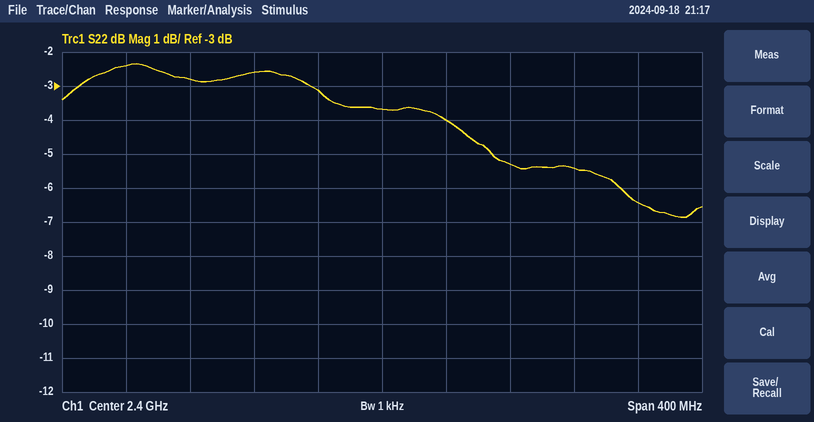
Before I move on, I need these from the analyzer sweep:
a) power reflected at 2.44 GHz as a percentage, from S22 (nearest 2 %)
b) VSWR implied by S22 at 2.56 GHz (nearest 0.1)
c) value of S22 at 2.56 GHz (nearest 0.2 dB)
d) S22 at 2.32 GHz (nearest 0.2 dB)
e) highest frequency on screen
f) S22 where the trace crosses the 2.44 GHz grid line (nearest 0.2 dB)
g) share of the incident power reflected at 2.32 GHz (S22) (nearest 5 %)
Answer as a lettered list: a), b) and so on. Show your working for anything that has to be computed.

a) 10^(-4/10) ≈ 40 %
b) |Γ| = 10^(-6.4/20) = 0.4786; VSWR = (1 + 0.4786)/(1 − 0.4786) ≈ 2.8
c) -6.4 dB
d) -2.6 dB
e) 2.6 GHz
f) -4.0 dB
g) 10^(-2.6/10) ≈ 55 %
